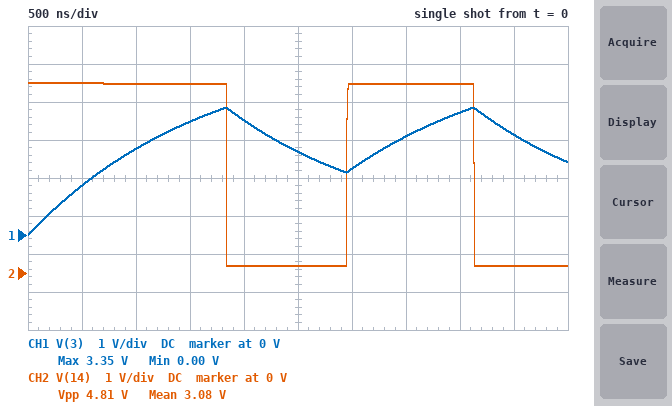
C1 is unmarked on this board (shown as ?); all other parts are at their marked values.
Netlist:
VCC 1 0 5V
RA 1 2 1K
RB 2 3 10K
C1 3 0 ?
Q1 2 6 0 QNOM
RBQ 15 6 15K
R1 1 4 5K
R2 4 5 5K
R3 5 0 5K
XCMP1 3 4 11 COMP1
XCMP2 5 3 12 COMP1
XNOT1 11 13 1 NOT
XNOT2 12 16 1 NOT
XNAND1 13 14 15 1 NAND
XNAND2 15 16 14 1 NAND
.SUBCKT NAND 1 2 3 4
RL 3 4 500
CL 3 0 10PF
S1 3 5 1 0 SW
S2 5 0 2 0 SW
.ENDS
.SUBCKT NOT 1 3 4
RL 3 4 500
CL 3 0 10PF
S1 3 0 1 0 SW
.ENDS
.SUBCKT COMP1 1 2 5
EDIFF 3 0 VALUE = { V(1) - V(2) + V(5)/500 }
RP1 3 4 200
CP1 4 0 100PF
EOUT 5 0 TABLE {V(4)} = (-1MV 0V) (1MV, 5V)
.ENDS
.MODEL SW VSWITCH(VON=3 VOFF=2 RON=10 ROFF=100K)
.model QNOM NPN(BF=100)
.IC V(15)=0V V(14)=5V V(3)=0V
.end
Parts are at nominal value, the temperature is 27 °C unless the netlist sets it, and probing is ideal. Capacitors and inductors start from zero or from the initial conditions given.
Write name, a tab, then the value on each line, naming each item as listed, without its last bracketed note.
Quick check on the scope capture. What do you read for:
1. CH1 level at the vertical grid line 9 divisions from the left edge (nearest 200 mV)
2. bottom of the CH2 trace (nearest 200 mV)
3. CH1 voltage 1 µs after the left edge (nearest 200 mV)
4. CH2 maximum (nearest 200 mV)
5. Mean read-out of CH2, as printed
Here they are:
CH1 level at the vertical grid line 9 divisions from the left edge	2.6 V
bottom of the CH2 trace	200 mV
CH1 voltage 1 µs after the left edge	2.2 V
CH2 maximum	5.0 V
Mean read-out of CH2, as printed	3.08 V
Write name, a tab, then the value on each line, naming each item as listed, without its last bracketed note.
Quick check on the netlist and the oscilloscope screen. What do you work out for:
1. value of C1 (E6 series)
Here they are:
value of C1	150 pF
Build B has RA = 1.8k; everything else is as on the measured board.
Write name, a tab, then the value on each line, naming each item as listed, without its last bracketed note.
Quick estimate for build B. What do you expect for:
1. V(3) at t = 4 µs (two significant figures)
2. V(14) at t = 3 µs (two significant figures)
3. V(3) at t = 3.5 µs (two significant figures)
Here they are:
V(3) at t = 4 µs	3.0 V
V(14) at t = 3 µs	190 mV
V(3) at t = 3.5 µs	2.4 V
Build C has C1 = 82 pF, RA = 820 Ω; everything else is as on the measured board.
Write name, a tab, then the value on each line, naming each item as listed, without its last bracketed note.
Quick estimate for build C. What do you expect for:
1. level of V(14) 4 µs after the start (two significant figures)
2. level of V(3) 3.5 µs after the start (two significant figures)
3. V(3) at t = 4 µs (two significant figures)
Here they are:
level of V(14) 4 µs after the start	190 mV
level of V(3) 3.5 µs after the start	3.3 V
V(3) at t = 4 µs	2.0 V
